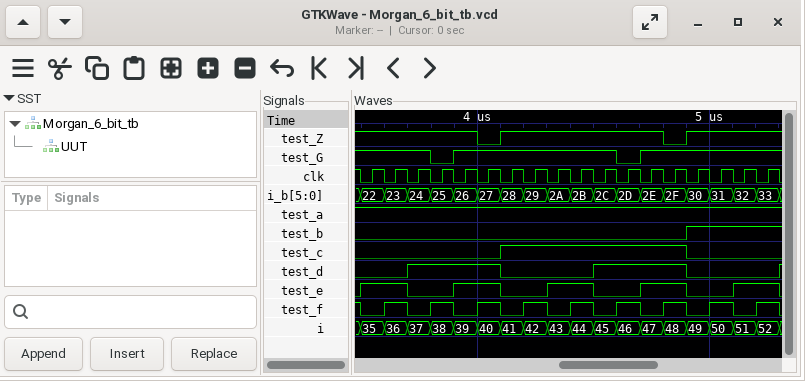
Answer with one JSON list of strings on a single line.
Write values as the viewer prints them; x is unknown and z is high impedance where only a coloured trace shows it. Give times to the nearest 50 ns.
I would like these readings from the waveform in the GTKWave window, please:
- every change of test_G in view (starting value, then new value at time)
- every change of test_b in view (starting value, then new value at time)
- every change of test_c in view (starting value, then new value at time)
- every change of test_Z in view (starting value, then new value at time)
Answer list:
["1, 0 at 3800 ns, 1 at 3900 ns, 0 at 4600 ns, 1 at 4700 ns", "0, 1 at 4900 ns", "0, 1 at 4100 ns, 0 at 4900 ns", "1, 0 at 4000 ns, 1 at 4100 ns, 0 at 4800 ns, 1 at 4900 ns"]
